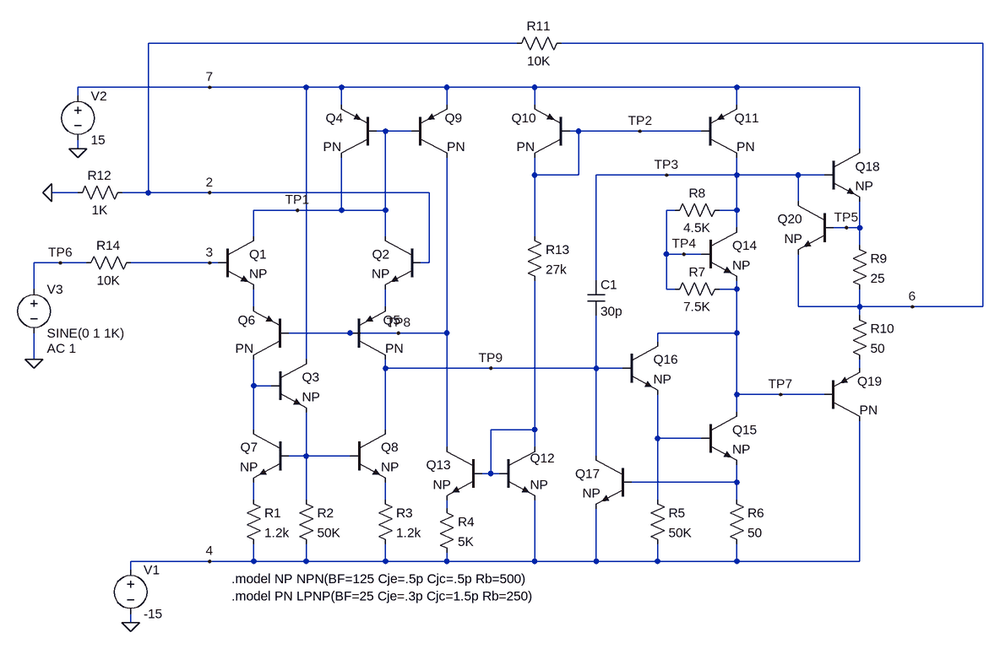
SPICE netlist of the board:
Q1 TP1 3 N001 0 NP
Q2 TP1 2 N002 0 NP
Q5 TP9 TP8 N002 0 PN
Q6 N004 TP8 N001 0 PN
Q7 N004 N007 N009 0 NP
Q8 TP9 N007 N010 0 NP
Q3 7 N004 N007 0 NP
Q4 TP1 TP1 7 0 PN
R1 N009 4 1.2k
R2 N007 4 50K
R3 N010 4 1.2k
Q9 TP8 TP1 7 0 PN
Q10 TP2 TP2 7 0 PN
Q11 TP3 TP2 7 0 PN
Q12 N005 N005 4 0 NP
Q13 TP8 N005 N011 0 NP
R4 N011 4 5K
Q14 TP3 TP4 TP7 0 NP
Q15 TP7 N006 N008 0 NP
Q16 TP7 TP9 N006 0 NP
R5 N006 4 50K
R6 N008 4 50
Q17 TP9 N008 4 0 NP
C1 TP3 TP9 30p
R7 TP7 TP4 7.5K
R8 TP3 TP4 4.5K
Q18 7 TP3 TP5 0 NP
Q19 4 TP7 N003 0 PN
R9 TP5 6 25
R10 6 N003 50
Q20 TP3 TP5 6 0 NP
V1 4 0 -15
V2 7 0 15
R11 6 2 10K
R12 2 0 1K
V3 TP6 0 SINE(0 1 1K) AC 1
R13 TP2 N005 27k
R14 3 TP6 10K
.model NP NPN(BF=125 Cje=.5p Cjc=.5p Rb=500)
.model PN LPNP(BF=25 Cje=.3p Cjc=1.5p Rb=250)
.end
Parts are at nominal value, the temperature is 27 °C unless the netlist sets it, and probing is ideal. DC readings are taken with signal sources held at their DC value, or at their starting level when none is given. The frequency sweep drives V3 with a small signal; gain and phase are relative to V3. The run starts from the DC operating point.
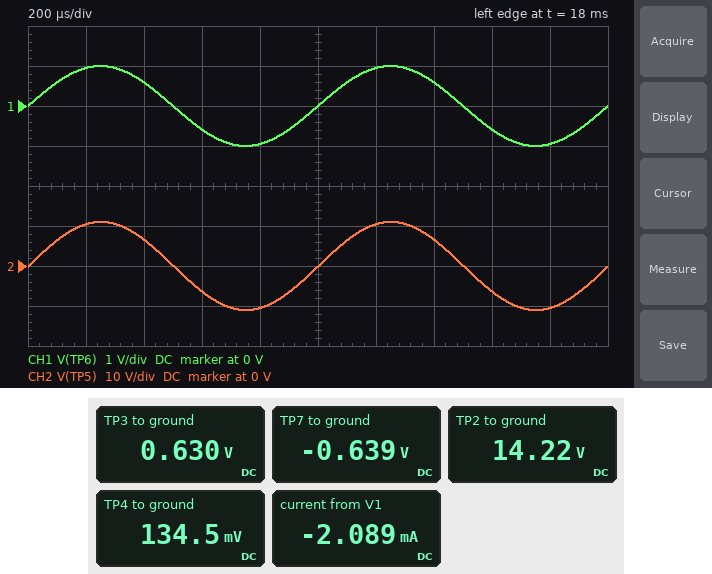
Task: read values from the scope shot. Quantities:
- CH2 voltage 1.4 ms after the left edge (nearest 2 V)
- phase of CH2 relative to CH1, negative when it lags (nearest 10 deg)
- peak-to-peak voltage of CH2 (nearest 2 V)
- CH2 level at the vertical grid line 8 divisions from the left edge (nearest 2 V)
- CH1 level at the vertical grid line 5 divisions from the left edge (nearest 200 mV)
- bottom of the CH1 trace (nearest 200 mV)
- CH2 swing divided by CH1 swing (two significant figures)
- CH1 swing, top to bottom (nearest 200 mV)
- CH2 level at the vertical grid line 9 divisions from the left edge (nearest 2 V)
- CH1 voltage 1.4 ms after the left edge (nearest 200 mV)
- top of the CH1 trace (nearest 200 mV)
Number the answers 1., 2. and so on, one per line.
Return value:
1. 6 V
2. 0 deg
3. 22 V
4. -6 V
5. 0 V
6. -1.0 V
7. 11
8. 2.0 V
9. -10 V
10. 600 mV
11. 1.0 V
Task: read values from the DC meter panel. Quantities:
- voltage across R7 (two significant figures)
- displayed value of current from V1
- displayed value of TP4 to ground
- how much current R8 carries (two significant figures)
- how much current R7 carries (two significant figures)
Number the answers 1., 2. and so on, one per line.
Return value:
1. 770 mV
2. -2.089 mA
3. 134.5 mV
4. 110 µA
5. 100 µA
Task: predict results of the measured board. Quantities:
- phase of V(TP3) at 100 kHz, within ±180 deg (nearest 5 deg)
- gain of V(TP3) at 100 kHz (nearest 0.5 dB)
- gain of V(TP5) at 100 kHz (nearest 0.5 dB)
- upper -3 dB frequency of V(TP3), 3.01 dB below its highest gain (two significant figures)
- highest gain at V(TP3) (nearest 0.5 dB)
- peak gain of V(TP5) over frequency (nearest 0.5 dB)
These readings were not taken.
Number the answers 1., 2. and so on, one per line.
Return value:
1. -55 deg
2. 18.5 dB
3. 16.5 dB
4. 77 kHz
5. 23.0 dB
6. 21.0 dB
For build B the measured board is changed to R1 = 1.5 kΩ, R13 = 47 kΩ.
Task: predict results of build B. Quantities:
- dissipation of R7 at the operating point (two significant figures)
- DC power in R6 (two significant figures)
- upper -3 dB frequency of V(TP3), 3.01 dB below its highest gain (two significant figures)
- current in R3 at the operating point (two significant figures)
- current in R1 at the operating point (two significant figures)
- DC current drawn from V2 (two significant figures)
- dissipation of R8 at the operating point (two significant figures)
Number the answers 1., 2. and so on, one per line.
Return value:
1. 76 µW
2. 15 µW
3. 62 kHz
4. 9.5 µA
5. 8.8 µA
6. 1.2 mA
7. 49 µW
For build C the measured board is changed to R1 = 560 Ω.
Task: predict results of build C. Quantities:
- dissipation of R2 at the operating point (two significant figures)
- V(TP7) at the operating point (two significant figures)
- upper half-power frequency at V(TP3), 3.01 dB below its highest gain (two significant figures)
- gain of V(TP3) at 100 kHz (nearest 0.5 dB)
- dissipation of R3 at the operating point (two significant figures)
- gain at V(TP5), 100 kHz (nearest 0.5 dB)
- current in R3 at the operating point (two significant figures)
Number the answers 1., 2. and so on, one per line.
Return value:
1. 8.8 µW
2. -770 mV
3. 70 kHz
4. 17.5 dB
5. 110 nW
6. 16.0 dB
7. 9.4 µA
